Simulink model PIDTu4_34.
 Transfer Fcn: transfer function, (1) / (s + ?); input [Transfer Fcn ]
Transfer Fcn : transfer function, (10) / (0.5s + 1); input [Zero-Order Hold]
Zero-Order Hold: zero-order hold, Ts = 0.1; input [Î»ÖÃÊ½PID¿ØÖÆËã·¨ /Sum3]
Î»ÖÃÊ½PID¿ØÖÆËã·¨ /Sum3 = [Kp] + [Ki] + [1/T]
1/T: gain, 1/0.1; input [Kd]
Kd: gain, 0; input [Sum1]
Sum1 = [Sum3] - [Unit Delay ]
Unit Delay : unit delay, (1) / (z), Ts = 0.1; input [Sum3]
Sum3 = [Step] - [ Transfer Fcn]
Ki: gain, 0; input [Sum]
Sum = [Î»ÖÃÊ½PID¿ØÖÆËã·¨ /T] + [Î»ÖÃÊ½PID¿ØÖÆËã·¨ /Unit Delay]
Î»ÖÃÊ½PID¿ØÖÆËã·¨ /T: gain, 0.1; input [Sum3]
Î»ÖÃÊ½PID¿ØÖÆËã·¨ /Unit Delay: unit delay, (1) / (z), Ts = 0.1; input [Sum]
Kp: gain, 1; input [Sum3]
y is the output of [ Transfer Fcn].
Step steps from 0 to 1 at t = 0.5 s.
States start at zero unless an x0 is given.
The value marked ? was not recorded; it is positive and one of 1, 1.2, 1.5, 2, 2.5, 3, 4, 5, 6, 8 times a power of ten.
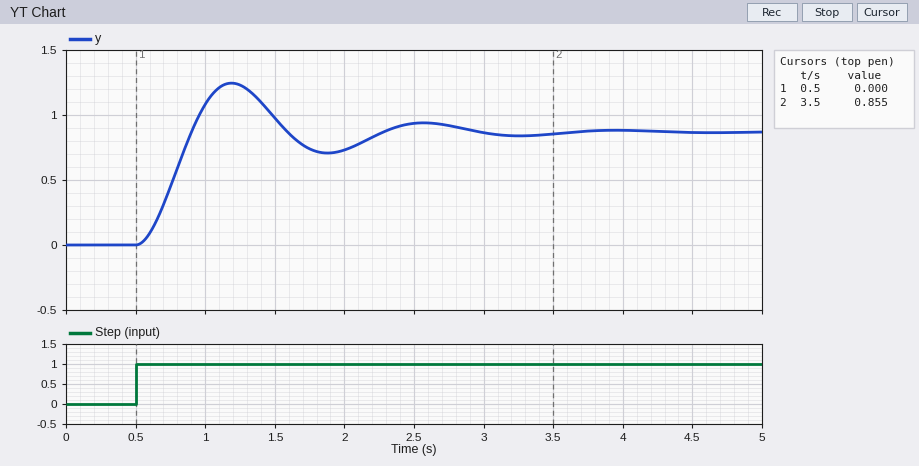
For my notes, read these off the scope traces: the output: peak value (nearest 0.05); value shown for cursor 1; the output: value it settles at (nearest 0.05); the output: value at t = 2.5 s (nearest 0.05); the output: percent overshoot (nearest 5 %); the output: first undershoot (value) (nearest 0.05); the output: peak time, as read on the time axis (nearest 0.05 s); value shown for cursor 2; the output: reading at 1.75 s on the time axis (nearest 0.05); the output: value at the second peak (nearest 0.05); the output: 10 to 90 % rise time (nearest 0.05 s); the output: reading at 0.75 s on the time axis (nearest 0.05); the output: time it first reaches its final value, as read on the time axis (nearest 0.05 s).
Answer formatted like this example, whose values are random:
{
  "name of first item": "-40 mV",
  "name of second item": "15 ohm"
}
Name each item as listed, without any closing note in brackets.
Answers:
{
  "the output: peak value": "1.25",
  "value shown for cursor 1": "0.000",
  "the output: value it settles at": "0.85",
  "the output: value at t = 2.5 s": "0.95",
  "the output: percent overshoot": "45 %",
  "the output: first undershoot (value)": "0.70",
  "the output: peak time, as read on the time axis": "1.20 s",
  "value shown for cursor 2": "0.855",
  "the output: reading at 1.75 s on the time axis": "0.75",
  "the output: value at the second peak": "0.95",
  "the output: 10 to 90 % rise time": "0.25 s",
  "the output: reading at 0.75 s on the time axis": "0.45",
  "the output: time it first reaches its final value, as read on the time axis": "0.90 s"
}
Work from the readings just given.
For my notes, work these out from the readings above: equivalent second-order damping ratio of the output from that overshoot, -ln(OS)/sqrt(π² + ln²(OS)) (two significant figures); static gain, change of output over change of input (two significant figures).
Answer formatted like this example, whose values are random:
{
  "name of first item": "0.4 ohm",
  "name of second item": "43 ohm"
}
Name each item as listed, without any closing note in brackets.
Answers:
{
  "equivalent second-order damping ratio of the output from that overshoot, -ln(OS)/sqrt(π² + ln²(OS))": "0.25",
  "static gain, change of output over change of input": "0.85"
}
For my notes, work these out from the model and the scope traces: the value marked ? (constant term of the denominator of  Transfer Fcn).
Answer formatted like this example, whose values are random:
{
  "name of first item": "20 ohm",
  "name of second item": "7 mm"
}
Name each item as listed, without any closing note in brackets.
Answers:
{
  "the value marked ?": "1.5"
}
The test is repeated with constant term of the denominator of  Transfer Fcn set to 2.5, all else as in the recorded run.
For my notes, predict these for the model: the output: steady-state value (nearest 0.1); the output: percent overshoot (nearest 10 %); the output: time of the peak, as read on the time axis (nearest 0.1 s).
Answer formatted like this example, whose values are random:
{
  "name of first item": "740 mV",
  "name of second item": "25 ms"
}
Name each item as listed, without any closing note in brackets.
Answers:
{
  "the output: steady-state value": "0.8",
  "the output: percent overshoot": "30 %",
  "the output: time of the peak, as read on the time axis": "1.2 s"
}
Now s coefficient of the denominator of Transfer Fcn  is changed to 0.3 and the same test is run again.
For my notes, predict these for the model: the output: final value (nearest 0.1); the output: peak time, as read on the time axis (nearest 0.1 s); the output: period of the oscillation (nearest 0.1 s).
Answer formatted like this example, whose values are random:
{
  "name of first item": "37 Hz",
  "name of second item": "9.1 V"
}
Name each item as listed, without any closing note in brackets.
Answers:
{
  "the output: final value": "0.9",
  "the output: peak time, as read on the time axis": "1.0 s",
  "the output: period of the oscillation": "1.1 s"
}
